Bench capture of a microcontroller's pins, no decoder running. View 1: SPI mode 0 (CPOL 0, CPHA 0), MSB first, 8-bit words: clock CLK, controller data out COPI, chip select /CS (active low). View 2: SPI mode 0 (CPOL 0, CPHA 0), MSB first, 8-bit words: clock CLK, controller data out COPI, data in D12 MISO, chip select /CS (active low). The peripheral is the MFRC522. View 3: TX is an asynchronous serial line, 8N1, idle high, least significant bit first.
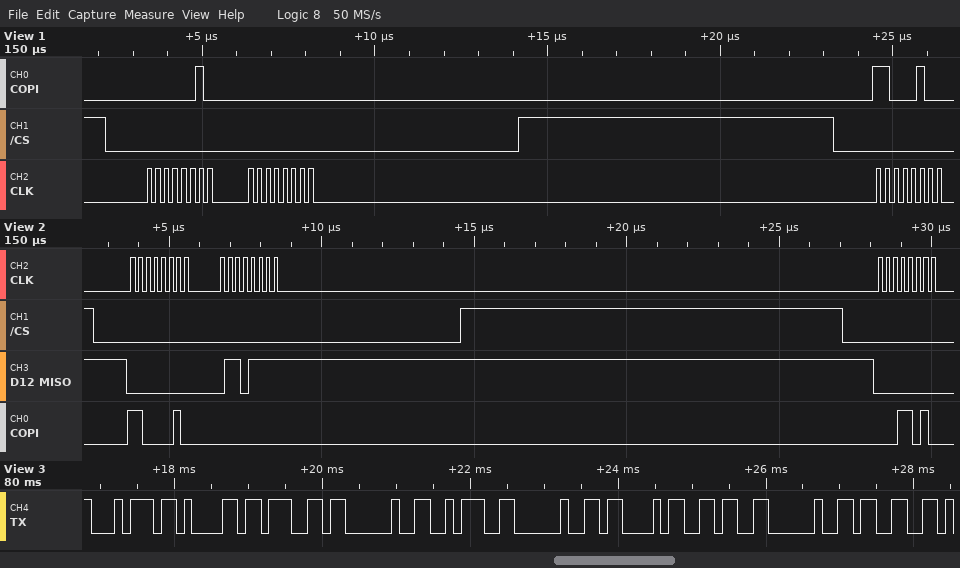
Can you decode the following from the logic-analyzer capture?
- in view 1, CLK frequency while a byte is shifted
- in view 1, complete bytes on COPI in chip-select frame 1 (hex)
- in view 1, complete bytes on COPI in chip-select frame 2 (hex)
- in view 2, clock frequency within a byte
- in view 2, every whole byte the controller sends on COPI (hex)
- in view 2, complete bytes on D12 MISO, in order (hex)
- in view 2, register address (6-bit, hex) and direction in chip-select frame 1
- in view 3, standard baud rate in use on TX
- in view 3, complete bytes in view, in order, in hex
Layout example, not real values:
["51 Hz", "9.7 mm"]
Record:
["4 MHz", "0x02 0x00", "0xC4", "4 MHz", "C2 00 1A", "00 6F 00", "0x21 read", "9600 baud", "74 61 67 20 3A 20 43 36 20 33"]
